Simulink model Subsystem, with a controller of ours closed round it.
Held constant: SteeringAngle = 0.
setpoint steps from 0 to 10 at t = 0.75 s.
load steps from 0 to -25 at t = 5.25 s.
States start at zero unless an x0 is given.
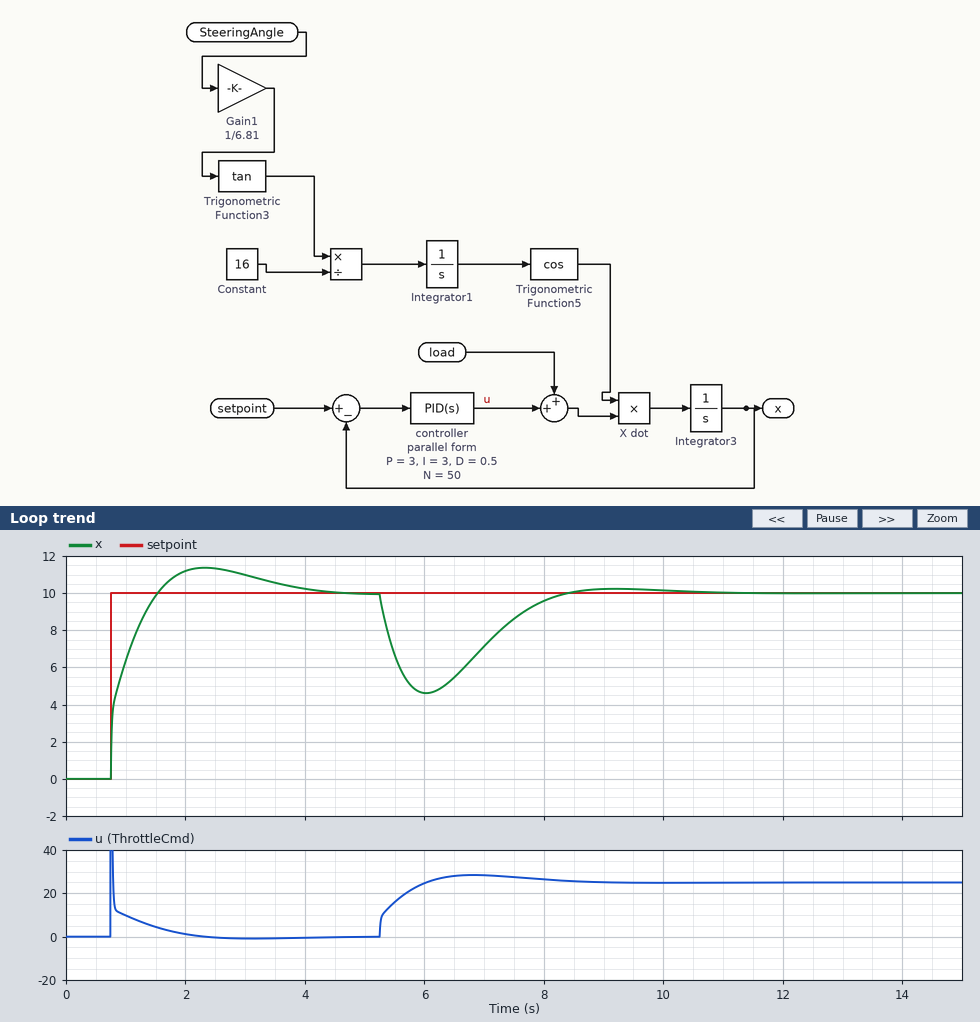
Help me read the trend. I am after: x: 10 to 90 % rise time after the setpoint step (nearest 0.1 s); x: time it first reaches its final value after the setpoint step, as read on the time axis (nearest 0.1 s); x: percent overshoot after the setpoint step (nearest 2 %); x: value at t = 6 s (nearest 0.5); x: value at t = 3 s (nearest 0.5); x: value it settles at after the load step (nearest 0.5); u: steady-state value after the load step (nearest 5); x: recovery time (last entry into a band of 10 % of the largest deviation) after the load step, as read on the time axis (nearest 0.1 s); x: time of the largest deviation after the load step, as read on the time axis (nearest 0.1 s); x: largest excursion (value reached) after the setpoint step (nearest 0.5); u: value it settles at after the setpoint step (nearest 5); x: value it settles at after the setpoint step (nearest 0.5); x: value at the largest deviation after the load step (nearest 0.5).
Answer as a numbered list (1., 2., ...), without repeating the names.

1. 0.6 s
2. 1.5 s
3. 14 %
4. 4.5
5. 11.0
6. 10.0
7. 25
8. 7.9 s
9. 6.0 s
10. 11.5
11. 0
12. 10.0
13. 4.5
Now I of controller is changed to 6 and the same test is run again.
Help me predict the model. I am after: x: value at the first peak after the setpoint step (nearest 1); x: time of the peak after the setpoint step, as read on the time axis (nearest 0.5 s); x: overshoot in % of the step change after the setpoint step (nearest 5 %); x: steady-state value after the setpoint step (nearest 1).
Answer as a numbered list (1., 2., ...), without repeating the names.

1. 12
2. 2.0 s
3. 20 %
4. 10
